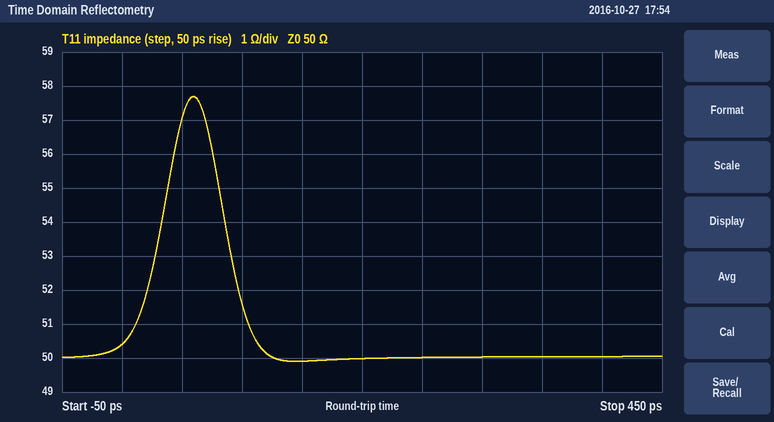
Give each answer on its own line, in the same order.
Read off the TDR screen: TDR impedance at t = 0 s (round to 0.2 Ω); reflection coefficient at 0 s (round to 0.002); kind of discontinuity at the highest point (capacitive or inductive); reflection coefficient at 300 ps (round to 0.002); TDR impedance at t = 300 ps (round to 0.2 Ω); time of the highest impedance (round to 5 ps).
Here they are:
50.4 Ω
+0.004
inductive
0.000
50.0 Ω
60 ps
